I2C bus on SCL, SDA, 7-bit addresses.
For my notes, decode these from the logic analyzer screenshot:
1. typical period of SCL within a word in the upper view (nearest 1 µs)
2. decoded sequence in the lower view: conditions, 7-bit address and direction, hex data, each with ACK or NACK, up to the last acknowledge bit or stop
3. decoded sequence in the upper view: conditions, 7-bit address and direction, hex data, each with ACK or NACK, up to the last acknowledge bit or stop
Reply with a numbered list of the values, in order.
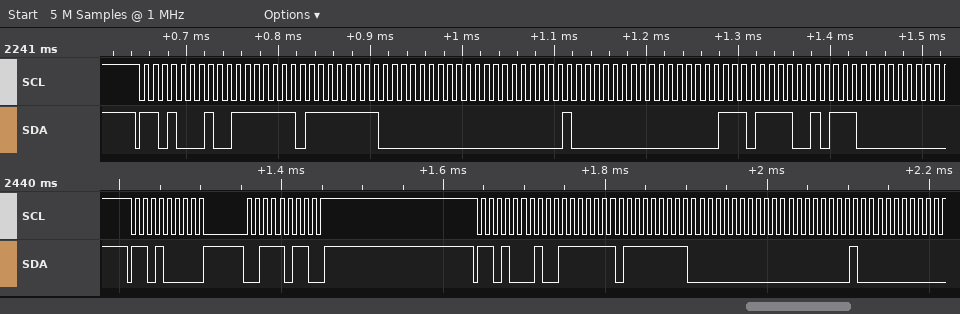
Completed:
1. 10 µs
2. start, address 68 write ACK, 3B ACK, stop, start, address 68 read ACK, 7F ACK, FF ACK, 00 ACK, 00 ACK, 40 ACK
3. start, address 68 read ACK, 7F ACK, FF ACK, 00 ACK, 00 ACK, 40 ACK, 00 ACK, EF ACK, 5C ACK
